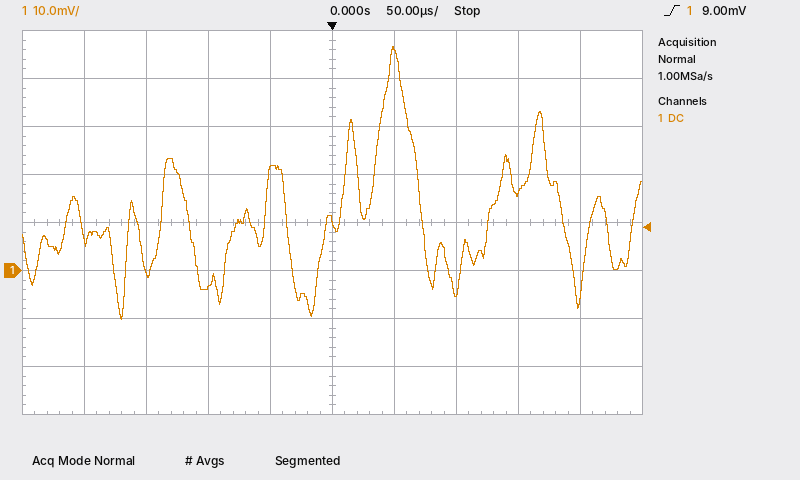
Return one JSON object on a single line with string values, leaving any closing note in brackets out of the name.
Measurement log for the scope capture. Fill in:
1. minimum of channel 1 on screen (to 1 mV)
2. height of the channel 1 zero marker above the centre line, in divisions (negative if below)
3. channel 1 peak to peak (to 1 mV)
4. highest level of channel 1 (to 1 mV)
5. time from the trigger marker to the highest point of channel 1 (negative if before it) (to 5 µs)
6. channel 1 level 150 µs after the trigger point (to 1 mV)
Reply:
{"minimum of channel 1 on screen": "-10 mV", "height of the channel 1 zero marker above the centre line, in divisions": "-1.0 div", "channel 1 peak to peak": "57 mV", "highest level of channel 1": "47 mV", "time from the trigger marker to the highest point of channel 1 (negative if before it)": "+50 µs", "channel 1 level 150 µs after the trigger point": "16 mV"}
